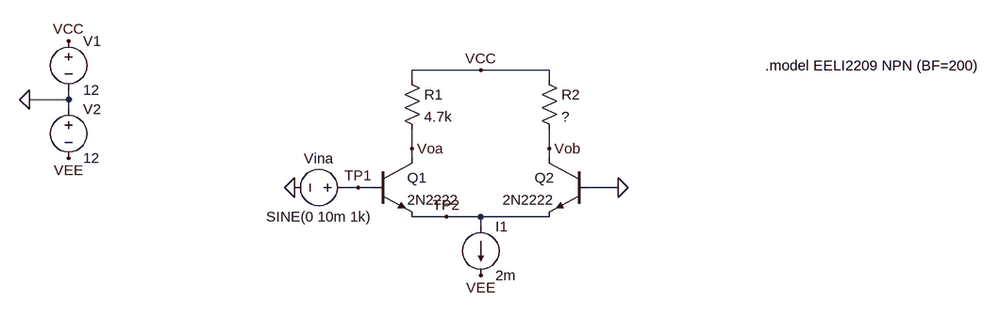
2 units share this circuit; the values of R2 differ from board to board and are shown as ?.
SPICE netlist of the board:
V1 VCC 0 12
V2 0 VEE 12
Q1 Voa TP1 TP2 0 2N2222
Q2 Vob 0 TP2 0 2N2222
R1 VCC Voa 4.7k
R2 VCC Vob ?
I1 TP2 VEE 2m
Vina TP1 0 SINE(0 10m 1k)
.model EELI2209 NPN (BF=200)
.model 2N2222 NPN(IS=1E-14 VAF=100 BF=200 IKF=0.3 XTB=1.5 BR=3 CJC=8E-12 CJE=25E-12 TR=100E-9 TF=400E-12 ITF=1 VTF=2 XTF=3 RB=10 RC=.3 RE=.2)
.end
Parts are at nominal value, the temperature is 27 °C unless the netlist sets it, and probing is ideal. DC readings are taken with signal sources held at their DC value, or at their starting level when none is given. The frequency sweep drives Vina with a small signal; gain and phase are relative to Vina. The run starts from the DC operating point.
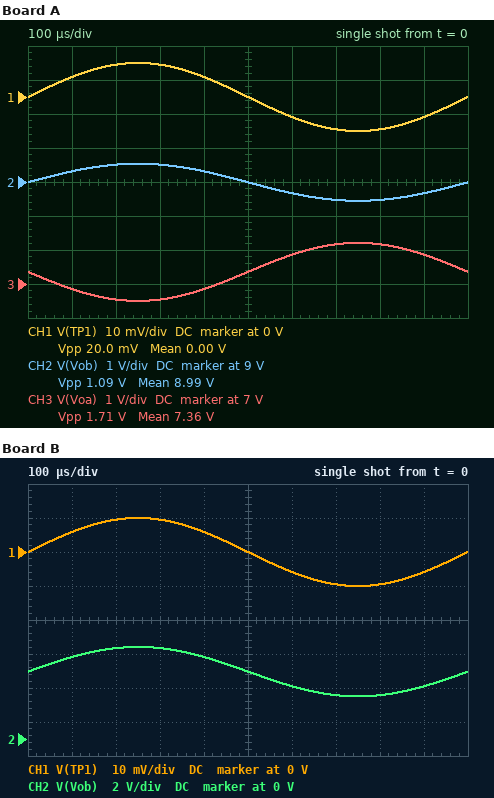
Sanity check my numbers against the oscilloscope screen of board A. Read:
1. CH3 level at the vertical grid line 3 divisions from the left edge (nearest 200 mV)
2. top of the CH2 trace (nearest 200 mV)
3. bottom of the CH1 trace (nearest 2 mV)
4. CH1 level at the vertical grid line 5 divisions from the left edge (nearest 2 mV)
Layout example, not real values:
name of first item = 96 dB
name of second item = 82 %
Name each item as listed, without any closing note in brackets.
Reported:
CH3 level at the vertical grid line 3 divisions from the left edge = 6.6 V
top of the CH2 trace = 9.6 V
bottom of the CH1 trace = -10 mV
CH1 level at the vertical grid line 5 divisions from the left edge = 0 V
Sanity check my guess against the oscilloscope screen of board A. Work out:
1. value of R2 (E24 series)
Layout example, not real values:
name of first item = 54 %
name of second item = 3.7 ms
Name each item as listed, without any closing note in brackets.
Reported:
value of R2 = 3 kΩ
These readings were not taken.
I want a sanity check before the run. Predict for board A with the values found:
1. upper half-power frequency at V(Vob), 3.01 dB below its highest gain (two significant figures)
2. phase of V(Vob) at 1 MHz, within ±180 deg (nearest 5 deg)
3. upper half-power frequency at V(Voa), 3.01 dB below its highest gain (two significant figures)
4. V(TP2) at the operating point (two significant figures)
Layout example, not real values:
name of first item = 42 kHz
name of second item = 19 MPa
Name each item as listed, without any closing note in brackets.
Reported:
upper half-power frequency at V(Vob), 3.01 dB below its highest gain = 11 MHz
phase of V(Vob) at 1 MHz, within ±180 deg = -5 deg
upper half-power frequency at V(Voa), 3.01 dB below its highest gain = 7.4 MHz
V(TP2) at the operating point = -650 mV
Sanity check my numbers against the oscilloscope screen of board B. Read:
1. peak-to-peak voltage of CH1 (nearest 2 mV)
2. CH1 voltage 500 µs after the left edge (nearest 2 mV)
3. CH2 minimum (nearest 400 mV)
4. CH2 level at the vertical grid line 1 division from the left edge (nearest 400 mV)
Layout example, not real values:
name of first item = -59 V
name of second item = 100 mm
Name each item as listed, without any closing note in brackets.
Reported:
peak-to-peak voltage of CH1 = 20 mV
CH1 voltage 500 µs after the left edge = 0 V
CH2 minimum = 2.4 V
CH2 level at the vertical grid line 1 division from the left edge = 4.8 V
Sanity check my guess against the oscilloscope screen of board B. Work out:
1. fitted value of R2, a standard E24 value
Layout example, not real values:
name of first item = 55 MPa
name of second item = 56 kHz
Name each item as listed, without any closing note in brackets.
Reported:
fitted value of R2, a standard E24 value = 8.2 kΩ
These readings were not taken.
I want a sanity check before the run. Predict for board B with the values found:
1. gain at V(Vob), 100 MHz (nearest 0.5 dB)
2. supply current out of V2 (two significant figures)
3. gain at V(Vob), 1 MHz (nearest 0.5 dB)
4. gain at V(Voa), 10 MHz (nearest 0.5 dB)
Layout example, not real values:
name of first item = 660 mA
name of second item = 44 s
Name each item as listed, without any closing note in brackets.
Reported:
gain at V(Vob), 100 MHz = 13.5 dB
supply current out of V2 = 2.0 mA
gain at V(Vob), 1 MHz = 43.0 dB
gain at V(Voa), 10 MHz = 33.5 dB
